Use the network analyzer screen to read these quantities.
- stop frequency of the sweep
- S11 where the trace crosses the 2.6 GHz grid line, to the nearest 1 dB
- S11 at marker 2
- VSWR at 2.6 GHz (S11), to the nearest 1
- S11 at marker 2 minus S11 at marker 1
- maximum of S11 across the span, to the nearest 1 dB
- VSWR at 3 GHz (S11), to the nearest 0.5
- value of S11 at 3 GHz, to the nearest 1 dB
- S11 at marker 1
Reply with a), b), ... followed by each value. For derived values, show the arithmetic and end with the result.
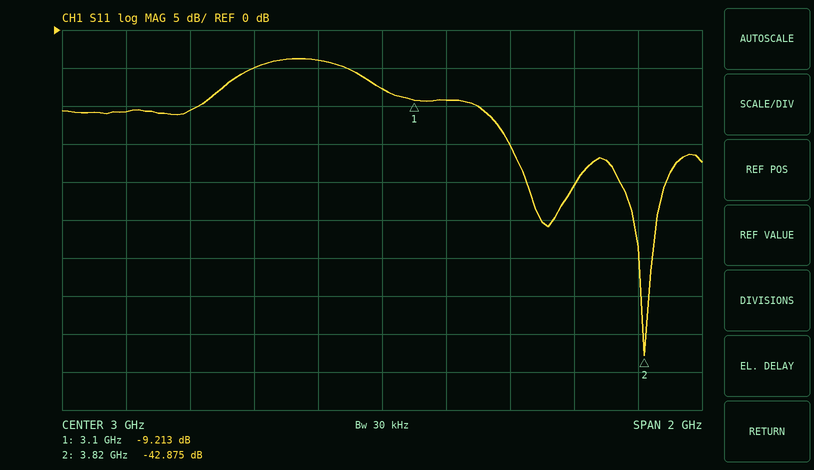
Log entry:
a) 4 GHz
b) -5 dB
c) -42.875 dB
d) |Γ| = 10^(-5/20) = 0.5623; VSWR = (1 + 0.5623)/(1 − 0.5623) ≈ 4
e) -42.875 − (-9.213) = -33.662 dB
f) -4 dB
g) |Γ| = 10^(-8/20) = 0.3981; VSWR = (1 + 0.3981)/(1 − 0.3981) ≈ 2.32, so 2.5 to the nearest 0.5
h) -8 dB
i) -9.213 dB
